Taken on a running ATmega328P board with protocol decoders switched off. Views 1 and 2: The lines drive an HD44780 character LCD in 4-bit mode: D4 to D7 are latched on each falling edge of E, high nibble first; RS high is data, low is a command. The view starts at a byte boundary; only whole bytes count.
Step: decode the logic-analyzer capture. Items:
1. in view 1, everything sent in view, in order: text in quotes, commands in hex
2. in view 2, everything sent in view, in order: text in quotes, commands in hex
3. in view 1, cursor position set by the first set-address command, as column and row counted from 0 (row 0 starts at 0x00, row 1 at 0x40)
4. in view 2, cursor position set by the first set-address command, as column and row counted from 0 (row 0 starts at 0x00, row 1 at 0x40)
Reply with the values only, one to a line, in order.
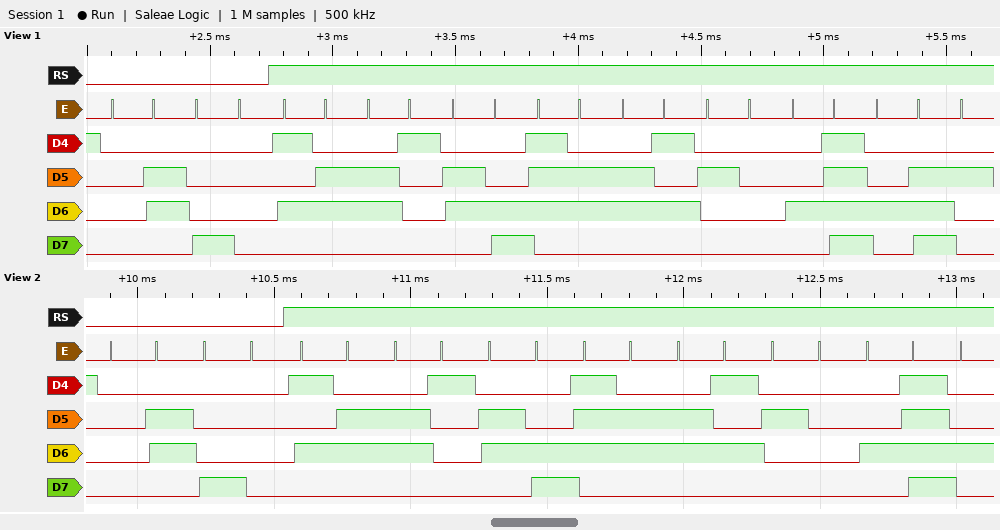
0x06 0x80 "Valve ON"
0x06 0x80 "Valve O"
column 0, row 0
column 0, row 0
